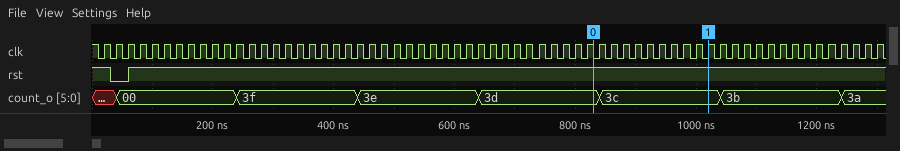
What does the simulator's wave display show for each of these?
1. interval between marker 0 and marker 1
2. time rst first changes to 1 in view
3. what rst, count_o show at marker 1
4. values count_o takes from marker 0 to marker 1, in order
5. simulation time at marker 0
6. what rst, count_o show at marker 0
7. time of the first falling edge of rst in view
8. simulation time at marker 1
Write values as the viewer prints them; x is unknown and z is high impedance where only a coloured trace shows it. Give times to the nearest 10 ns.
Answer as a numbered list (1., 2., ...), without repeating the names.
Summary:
1. 190 ns
2. 60 ns
3. rst=1, count_o=3c
4. 3d, 3c
5. 830 ns
6. rst=1, count_o=3d
7. 30 ns
8. 1020 ns
